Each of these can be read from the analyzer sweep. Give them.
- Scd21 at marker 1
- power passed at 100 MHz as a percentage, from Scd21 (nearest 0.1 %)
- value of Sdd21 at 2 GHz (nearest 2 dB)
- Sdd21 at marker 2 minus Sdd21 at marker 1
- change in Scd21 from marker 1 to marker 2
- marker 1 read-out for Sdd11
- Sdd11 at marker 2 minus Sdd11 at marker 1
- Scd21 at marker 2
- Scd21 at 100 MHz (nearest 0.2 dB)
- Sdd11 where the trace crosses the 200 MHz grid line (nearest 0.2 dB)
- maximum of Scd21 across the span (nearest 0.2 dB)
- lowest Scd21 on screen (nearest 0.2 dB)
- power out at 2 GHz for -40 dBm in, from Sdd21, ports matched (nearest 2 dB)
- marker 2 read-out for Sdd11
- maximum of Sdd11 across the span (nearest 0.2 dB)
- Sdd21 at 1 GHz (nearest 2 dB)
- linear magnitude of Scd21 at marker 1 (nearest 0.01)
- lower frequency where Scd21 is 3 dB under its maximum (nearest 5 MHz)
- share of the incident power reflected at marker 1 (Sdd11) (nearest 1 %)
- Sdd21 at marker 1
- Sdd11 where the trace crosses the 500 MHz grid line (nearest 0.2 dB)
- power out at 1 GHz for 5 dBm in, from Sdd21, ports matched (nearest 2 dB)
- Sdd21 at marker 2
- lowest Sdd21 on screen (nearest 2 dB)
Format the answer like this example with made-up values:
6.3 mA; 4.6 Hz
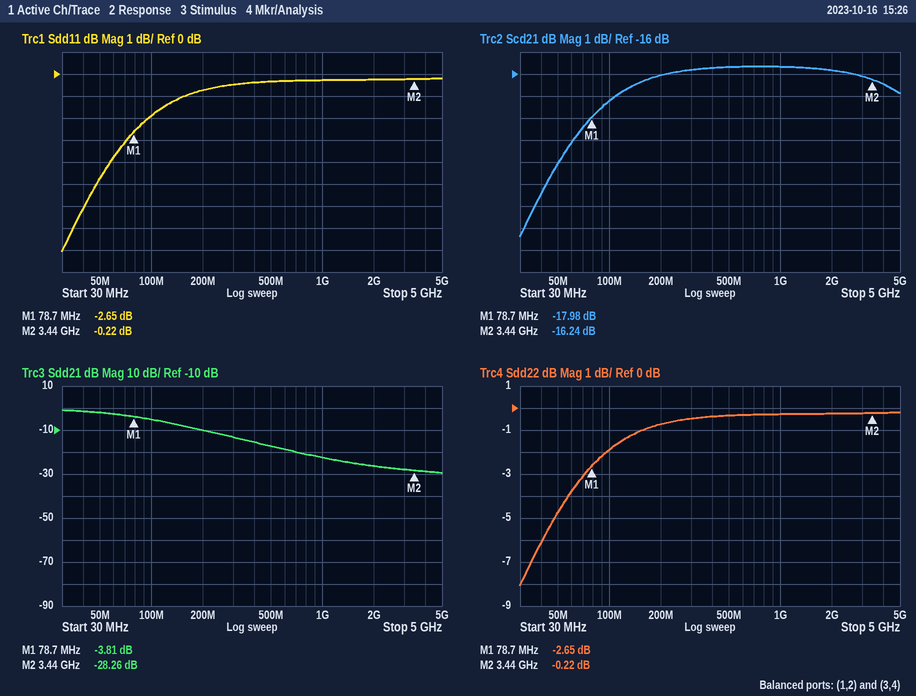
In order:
-17.98 dB; 1.9 %; -26 dB; -24.45 dB; 1.74 dB; -2.65 dB; 2.43 dB; -16.24 dB; -17.2 dB; -0.8 dB; -15.6 dB; -23.4 dB; -66 dBm; -0.22 dB; -0.2 dB; -22 dB; 0.13; 65 MHz; 54 %; -3.81 dB; -0.4 dB; -18 dBm; -28.26 dB; -30 dB
